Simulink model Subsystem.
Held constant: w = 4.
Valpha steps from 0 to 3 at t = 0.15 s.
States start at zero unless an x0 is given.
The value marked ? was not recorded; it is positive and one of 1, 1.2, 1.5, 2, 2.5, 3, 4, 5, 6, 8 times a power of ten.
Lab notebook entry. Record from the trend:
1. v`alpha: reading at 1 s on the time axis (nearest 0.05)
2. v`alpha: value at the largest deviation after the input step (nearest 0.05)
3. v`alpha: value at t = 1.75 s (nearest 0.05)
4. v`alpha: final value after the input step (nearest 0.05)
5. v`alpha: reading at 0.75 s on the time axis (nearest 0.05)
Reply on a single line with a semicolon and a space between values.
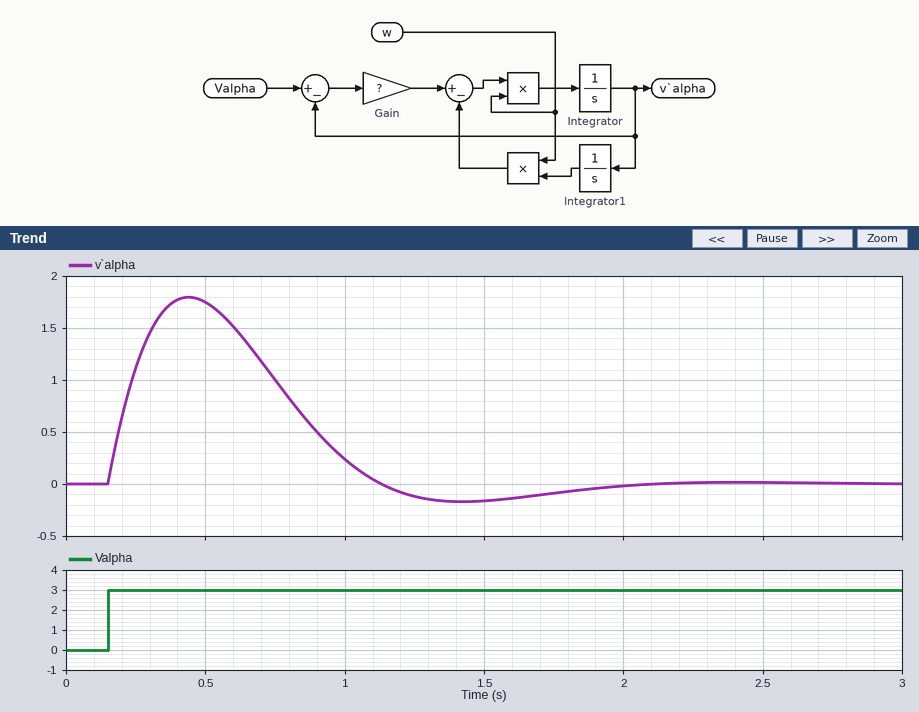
0.25; 1.80; -0.10; 0.00; 1.00
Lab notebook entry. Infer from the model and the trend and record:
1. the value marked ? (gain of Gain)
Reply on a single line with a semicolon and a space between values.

1.2
